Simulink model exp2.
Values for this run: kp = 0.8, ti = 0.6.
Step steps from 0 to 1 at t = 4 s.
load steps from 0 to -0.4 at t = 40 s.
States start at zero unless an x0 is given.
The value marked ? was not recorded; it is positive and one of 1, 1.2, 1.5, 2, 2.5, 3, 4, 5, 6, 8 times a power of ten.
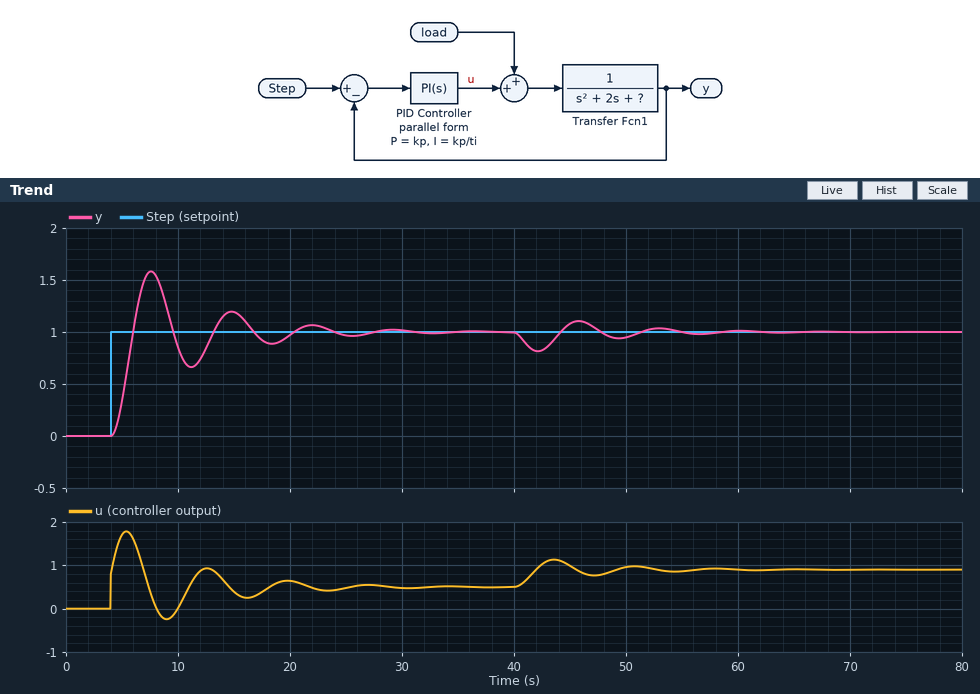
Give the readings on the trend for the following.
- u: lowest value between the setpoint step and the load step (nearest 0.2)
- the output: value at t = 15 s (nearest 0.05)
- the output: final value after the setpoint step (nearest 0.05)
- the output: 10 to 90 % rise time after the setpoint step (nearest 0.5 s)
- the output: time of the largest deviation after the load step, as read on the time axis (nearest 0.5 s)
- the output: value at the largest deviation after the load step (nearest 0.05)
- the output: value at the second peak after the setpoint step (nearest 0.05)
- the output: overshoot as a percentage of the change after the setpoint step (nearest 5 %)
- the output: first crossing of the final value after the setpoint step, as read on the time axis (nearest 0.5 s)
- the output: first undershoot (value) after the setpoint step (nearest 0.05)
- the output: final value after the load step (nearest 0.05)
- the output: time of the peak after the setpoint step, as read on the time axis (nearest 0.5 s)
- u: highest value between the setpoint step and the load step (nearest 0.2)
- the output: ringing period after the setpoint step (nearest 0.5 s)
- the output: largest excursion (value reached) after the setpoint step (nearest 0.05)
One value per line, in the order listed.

-0.2
1.20
1.00
1.5 s
42.0 s
0.80
1.20
60 %
6.0 s
0.65
1.00
7.5 s
1.8
7.0 s
1.60
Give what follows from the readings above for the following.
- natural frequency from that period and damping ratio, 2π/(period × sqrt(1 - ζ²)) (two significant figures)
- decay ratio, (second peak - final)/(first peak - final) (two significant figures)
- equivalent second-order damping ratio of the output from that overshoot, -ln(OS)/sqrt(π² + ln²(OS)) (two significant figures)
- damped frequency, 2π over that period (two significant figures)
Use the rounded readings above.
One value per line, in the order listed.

0.91 rad/s
0.33
0.16
0.90 rad/s
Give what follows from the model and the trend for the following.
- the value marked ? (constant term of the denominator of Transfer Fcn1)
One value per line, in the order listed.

0.5
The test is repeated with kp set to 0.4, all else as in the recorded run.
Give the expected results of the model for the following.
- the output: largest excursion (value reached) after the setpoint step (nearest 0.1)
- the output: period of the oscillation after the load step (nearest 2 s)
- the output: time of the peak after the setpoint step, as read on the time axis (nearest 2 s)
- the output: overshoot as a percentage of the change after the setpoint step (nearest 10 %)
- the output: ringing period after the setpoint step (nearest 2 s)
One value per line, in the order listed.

1.5
10 s
10 s
50 %
10 s
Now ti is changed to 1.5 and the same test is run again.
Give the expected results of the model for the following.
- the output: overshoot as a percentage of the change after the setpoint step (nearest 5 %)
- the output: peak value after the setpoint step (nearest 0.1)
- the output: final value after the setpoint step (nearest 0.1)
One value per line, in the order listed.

20 %
1.2
1.0
